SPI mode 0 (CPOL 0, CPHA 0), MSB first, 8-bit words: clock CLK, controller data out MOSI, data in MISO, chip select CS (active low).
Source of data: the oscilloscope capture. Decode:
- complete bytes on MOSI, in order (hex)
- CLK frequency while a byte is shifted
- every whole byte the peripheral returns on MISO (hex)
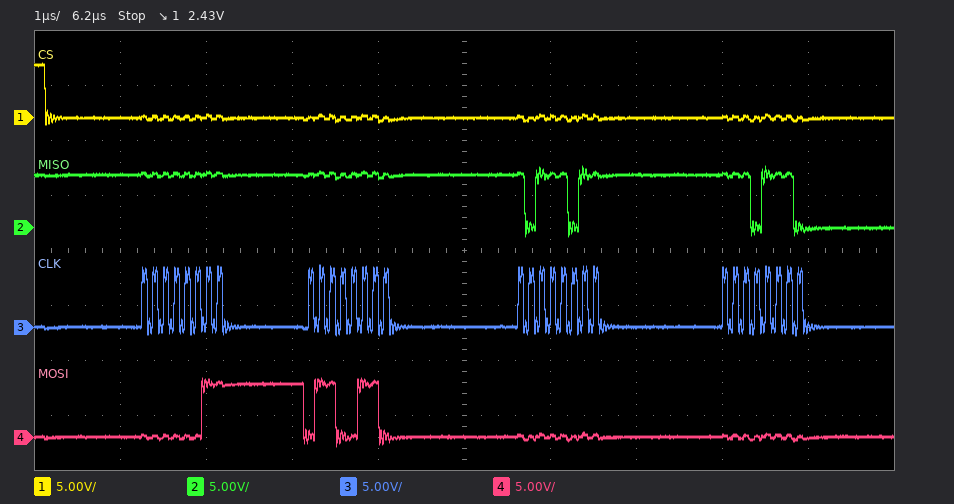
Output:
03 66 00 00
8 MHz
FF FF BB EE
